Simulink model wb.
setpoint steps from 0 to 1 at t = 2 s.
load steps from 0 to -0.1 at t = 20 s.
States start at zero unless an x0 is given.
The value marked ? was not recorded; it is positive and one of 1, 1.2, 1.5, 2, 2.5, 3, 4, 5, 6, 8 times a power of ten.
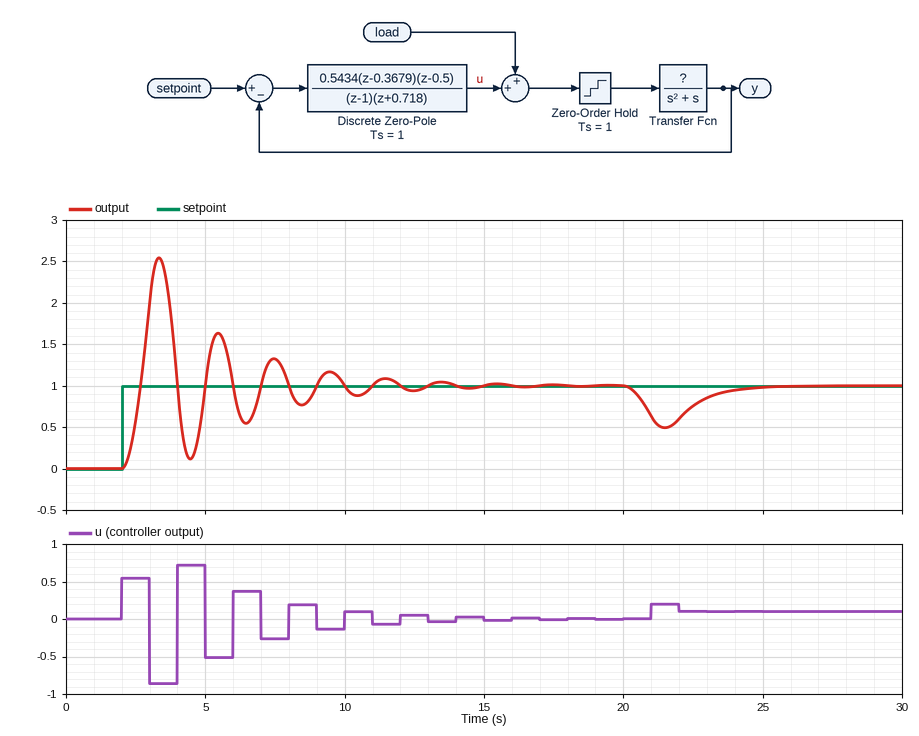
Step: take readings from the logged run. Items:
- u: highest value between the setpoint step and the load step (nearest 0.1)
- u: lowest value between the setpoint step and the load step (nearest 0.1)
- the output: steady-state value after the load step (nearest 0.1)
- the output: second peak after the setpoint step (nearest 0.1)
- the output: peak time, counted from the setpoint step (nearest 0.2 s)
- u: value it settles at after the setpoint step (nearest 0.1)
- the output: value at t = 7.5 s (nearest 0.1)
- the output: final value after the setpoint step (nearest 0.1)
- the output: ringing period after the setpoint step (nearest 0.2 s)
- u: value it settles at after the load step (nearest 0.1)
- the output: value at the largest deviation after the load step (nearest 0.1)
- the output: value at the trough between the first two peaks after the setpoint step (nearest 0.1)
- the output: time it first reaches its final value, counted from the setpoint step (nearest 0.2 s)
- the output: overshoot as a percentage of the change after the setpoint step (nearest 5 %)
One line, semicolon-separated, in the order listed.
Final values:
0.7; -0.9; 1.0; 1.6; 1.4 s; 0.0; 1.3; 1.0; 2.2 s; 0.1; 0.5; 0.1; 0.6 s; 155 %
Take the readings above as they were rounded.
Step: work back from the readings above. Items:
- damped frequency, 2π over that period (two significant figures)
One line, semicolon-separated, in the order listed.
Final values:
2.9 rad/s
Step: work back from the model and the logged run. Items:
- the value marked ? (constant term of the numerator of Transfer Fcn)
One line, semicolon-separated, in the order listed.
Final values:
10
